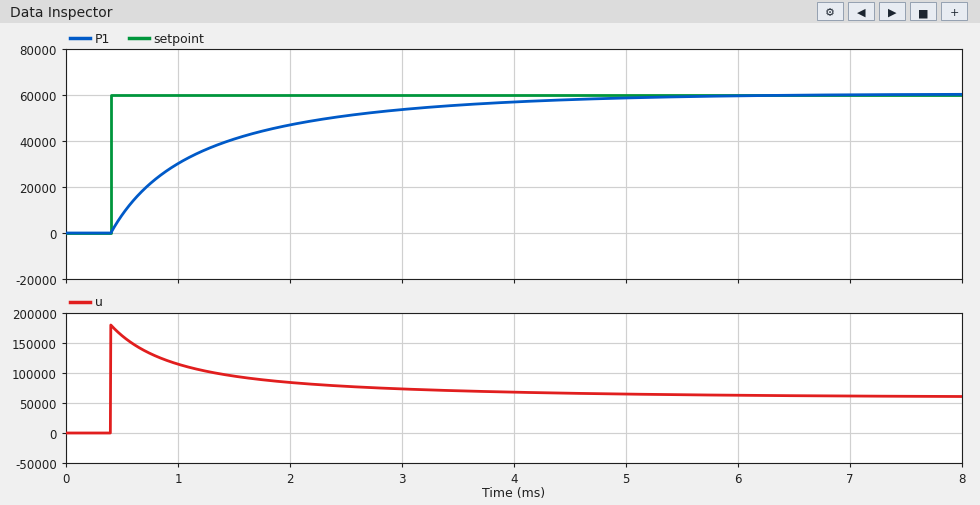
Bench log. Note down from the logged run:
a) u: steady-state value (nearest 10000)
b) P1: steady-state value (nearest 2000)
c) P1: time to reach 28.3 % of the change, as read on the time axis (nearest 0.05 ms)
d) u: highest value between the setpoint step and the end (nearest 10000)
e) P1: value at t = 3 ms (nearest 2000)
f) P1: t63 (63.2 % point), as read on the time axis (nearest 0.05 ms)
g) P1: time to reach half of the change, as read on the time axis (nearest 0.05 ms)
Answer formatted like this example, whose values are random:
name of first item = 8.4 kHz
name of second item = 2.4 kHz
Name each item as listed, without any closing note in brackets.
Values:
u: steady-state value = 60000
P1: steady-state value = 60000
P1: time to reach 28.3 % of the change, as read on the time axis = 0.65 ms
u: highest value between the setpoint step and the end = 180000
P1: value at t = 3 ms = 54000
P1: t63 (63.2 % point), as read on the time axis = 1.35 ms
P1: time to reach half of the change, as read on the time axis = 1.00 ms
